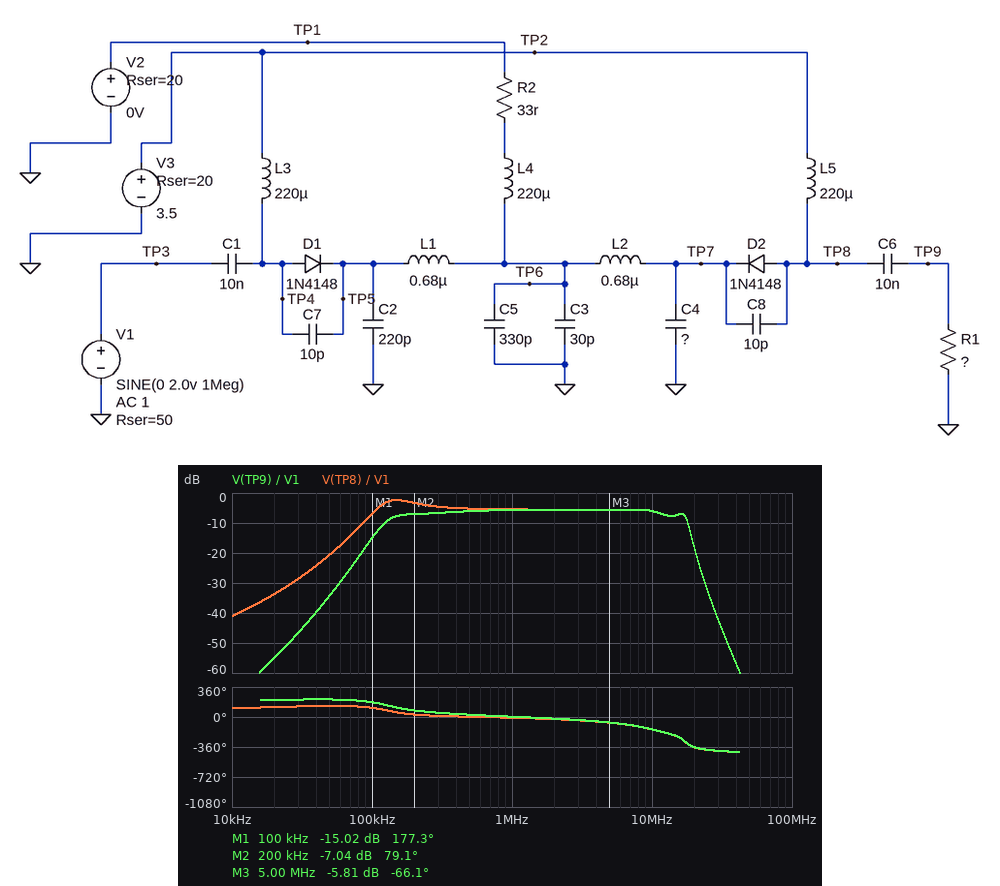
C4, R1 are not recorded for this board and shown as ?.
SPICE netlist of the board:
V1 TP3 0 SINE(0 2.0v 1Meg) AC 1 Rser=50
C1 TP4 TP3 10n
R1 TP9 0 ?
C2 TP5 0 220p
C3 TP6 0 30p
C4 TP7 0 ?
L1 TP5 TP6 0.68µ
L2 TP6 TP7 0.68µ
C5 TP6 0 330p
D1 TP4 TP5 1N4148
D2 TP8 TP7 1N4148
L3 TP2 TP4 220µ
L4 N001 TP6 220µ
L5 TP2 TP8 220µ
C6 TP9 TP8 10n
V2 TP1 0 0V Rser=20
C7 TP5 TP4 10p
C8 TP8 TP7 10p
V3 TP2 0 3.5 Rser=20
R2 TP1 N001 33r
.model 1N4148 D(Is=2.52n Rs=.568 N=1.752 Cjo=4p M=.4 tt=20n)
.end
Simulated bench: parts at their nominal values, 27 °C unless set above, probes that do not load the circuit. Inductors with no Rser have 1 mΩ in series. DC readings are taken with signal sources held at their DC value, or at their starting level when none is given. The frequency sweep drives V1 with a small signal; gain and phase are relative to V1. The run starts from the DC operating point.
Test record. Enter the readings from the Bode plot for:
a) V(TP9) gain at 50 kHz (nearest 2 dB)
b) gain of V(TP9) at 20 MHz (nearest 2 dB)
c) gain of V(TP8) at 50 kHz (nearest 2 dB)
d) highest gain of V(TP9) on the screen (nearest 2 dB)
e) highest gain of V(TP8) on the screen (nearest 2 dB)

-34 dB
-18 dB
-20 dB
-6 dB
-2 dB
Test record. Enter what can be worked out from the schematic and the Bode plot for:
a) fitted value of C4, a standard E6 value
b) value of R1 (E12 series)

470 pF
68 Ω
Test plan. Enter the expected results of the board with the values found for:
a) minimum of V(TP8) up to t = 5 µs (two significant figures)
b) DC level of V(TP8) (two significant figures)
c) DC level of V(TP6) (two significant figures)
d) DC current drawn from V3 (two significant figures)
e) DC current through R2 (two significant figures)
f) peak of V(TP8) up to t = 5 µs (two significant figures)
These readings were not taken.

1.6 V
2.7 V
2.0 V
38 mA
38 mA
3.8 V
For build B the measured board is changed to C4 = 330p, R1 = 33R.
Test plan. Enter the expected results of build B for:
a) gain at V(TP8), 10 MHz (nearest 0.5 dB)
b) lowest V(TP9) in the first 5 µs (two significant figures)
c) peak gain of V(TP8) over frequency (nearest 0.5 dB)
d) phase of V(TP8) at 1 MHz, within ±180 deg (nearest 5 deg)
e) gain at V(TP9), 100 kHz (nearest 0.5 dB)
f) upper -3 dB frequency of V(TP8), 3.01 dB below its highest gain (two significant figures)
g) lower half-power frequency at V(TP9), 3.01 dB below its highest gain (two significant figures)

-8.5 dB
-660 mV
-1.0 dB
-15 deg
-20.0 dB
220 kHz
290 kHz
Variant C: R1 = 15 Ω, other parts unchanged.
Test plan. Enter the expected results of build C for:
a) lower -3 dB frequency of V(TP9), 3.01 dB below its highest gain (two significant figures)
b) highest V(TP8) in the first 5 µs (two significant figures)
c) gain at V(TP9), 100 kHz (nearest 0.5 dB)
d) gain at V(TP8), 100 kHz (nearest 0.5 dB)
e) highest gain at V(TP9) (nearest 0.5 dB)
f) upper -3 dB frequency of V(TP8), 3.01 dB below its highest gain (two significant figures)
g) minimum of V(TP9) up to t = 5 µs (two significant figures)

470 kHz
3.3 V
-26.0 dB
-5.5 dB
-13.0 dB
200 kHz
-320 mV
